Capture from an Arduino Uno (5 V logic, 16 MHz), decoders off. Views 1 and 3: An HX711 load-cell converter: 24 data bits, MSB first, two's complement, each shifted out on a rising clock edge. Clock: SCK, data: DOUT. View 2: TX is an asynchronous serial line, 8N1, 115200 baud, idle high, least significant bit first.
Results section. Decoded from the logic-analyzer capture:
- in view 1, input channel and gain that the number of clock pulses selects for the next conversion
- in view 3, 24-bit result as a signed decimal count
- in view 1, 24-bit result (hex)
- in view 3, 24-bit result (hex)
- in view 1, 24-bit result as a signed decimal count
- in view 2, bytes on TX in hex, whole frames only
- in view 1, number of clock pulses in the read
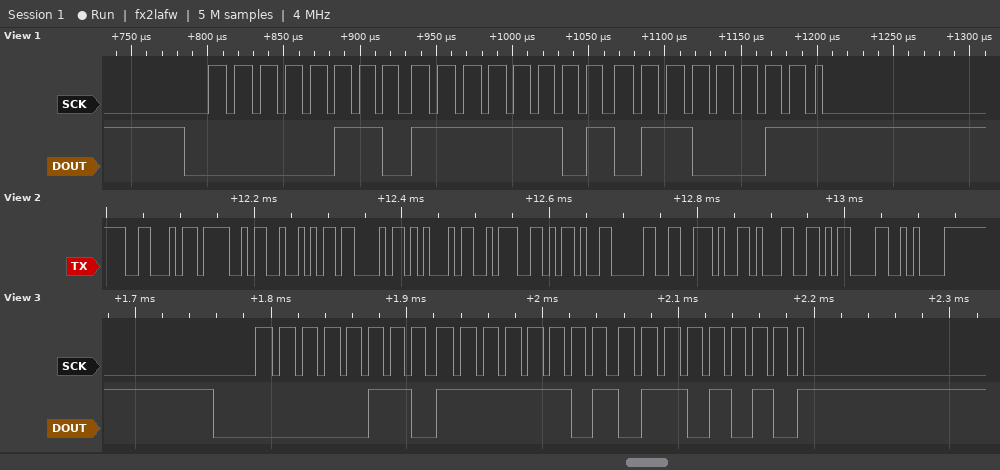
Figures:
channel A, gain 128
458090
0x06FD63
0x06FD6A
458083
46 4F 52 43 45 3A 2D 30 2E 31 0D 0A
25
